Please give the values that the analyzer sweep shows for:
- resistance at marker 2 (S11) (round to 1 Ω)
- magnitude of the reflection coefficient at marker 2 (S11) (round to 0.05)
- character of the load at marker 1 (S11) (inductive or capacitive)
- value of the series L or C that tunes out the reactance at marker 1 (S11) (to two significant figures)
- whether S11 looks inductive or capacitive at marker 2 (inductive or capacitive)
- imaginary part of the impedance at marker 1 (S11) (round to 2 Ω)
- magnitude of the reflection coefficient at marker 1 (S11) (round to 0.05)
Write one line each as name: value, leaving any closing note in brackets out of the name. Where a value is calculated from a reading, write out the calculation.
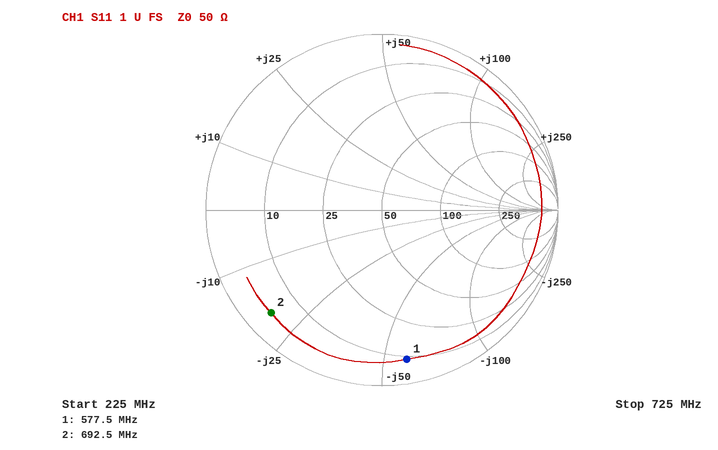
resistance at marker 2 (S11): 4 Ω
magnitude of the reflection coefficient at marker 2 (S11): 0.85
character of the load at marker 1 (S11): capacitive
value of the series L or C that tunes out the reactance at marker 1 (S11): L = 58 Ω/(2π × 577.5 MHz) ≈ 16 nH
whether S11 looks inductive or capacitive at marker 2: capacitive
imaginary part of the impedance at marker 1 (S11): -58 Ω
magnitude of the reflection coefficient at marker 1 (S11): 0.85
